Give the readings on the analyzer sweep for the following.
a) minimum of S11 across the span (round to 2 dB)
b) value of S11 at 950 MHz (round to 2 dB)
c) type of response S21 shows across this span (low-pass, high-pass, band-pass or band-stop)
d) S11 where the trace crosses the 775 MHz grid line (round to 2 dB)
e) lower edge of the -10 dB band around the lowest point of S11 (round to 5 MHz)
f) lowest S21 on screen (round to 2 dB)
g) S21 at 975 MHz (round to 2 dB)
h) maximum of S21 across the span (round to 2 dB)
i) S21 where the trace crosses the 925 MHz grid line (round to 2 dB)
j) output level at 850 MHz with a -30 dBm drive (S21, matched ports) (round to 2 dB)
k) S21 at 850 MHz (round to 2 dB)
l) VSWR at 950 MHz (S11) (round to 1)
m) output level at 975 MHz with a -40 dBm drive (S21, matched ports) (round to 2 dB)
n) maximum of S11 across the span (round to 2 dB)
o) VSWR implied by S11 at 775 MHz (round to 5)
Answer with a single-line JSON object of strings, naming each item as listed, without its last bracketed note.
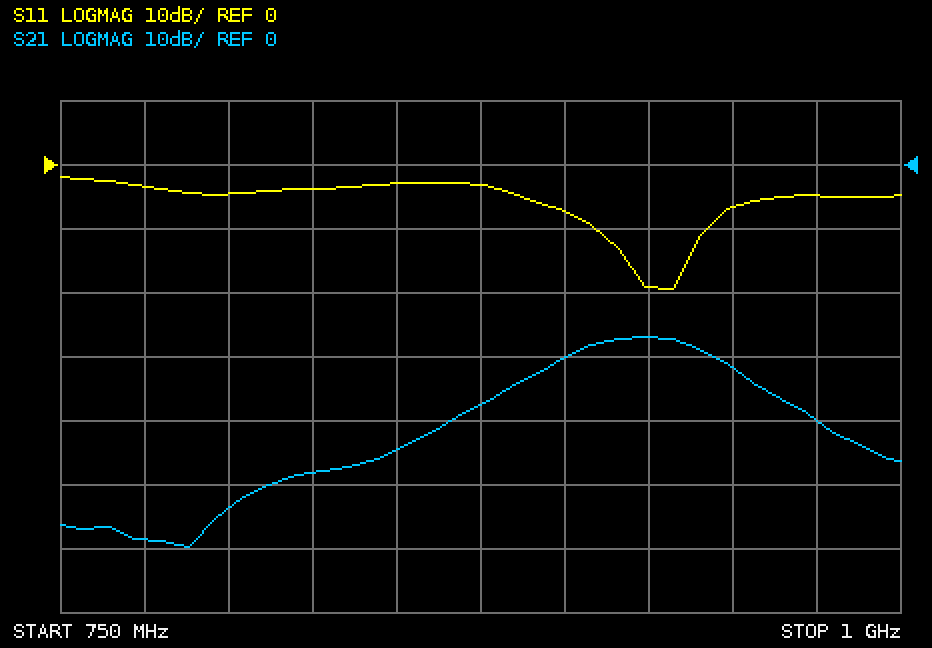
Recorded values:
{"minimum of S11 across the span": "-20 dB", "value of S11 at 950 MHz": "-6 dB", "type of response S21 shows across this span": "band-pass", "S11 where the trace crosses the 775 MHz grid line": "-4 dB", "lower edge of the -10 dB band around the lowest point of S11": "910 MHz", "lowest S21 on screen": "-60 dB", "S21 at 975 MHz": "-40 dB", "maximum of S21 across the span": "-26 dB", "S21 where the trace crosses the 925 MHz grid line": "-26 dB", "output level at 850 MHz with a -30 dBm drive (S21, matched ports)": "-74 dBm", "S21 at 850 MHz": "-44 dB", "VSWR at 950 MHz (S11)": "3", "output level at 975 MHz with a -40 dBm drive (S21, matched ports)": "-80 dBm", "maximum of S11 across the span": "-2 dB", "VSWR implied by S11 at 775 MHz": "5"}
